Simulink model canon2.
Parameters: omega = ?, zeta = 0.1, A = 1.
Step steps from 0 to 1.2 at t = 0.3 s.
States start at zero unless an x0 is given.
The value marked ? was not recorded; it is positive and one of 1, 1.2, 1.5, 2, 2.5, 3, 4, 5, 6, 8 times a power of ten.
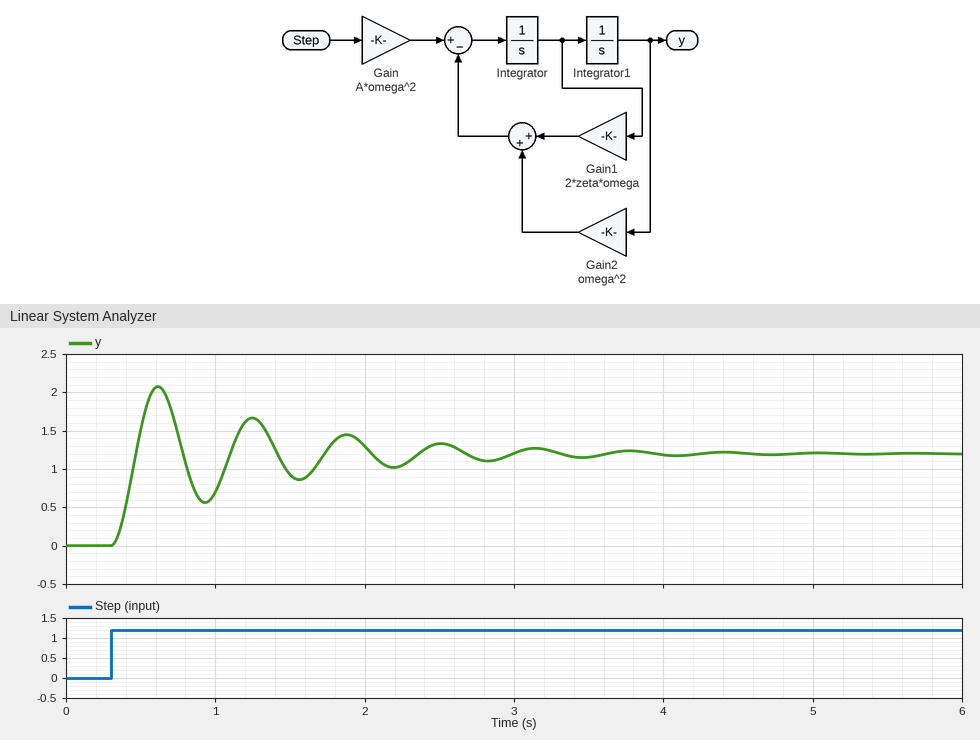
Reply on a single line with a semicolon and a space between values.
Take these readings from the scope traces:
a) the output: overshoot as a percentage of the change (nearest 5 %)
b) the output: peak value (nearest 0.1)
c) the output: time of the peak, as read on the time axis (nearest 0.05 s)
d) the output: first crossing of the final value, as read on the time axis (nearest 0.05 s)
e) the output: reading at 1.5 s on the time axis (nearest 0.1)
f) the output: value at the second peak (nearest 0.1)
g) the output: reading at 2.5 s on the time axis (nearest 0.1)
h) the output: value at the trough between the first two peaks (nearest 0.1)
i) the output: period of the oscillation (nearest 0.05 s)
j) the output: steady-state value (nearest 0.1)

75 %; 2.1; 0.60 s; 0.45 s; 0.9; 1.7; 1.3; 0.6; 0.65 s; 1.2
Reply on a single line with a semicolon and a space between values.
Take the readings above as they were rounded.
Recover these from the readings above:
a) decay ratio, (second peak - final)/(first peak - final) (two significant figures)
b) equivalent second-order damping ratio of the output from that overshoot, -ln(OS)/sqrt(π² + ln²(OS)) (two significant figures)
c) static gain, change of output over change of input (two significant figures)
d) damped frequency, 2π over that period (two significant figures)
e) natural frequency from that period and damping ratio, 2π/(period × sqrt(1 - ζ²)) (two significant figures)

0.56; 0.091; 1.0; 9.7 rad/s; 9.7 rad/s
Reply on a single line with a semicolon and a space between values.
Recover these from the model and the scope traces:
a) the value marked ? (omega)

10
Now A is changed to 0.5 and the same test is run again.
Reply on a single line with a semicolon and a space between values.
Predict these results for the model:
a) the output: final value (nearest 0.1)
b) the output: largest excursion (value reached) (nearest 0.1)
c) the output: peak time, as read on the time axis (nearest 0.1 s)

0.6; 1.0; 0.6 s
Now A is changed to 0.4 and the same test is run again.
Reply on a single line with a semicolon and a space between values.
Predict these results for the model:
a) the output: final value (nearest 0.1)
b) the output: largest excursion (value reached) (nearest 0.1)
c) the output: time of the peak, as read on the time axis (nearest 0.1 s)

0.5; 0.8; 0.6 s
